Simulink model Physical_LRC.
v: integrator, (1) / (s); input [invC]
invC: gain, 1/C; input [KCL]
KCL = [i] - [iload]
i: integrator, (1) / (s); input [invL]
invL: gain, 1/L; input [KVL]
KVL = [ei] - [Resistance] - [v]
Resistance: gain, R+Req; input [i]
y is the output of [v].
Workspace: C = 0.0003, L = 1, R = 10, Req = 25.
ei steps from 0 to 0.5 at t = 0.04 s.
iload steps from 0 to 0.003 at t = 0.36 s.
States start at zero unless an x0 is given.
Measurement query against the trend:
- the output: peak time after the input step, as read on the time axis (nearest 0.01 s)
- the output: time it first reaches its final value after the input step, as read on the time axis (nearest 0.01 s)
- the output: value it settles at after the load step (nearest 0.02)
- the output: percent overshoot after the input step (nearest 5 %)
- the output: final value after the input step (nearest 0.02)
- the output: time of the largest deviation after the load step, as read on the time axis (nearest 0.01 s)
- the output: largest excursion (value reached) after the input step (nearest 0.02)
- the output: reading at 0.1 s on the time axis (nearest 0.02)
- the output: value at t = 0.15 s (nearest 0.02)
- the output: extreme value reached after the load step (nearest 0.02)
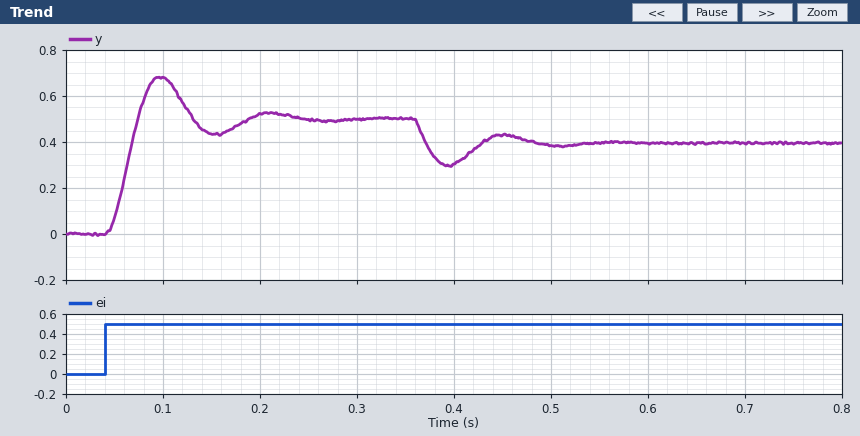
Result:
0.10 s
0.07 s
0.40
35 %
0.50
0.39 s
0.68
0.68
0.44
0.30
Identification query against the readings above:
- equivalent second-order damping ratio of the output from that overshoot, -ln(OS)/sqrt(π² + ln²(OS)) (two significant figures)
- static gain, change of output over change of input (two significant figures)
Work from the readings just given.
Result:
0.32
1.0
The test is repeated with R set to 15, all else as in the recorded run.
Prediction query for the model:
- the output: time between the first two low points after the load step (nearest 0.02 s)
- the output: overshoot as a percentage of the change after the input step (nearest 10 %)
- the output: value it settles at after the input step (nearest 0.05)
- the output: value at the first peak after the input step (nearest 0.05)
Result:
0.12 s
30 %
0.50
0.65
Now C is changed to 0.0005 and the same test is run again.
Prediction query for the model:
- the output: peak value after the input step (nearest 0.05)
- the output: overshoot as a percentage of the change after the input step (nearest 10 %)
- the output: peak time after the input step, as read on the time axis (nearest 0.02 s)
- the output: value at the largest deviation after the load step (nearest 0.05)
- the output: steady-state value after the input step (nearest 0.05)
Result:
0.65
30 %
0.12 s
0.35
0.50
